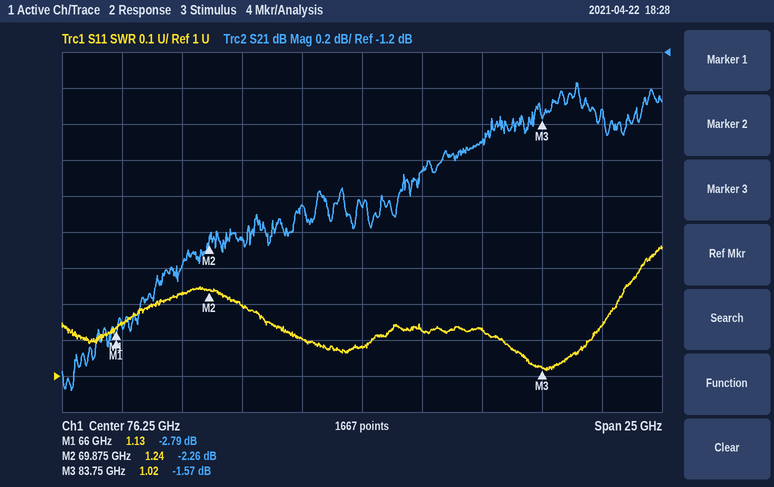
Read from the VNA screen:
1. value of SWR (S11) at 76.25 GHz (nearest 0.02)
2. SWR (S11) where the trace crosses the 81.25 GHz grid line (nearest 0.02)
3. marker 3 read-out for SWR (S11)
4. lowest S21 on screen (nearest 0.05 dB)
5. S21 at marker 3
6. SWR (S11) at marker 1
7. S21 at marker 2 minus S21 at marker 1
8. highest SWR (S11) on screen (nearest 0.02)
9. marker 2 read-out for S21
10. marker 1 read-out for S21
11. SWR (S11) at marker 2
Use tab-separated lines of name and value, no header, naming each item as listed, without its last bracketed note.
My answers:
value of SWR (S11) at 76.25 GHz	1.08
SWR (S11) where the trace crosses the 81.25 GHz grid line	1.14
marker 3 read-out for SWR	1.02
lowest S21 on screen	-3.10 dB
S21 at marker 3	-1.57 dB
SWR (S11) at marker 1	1.13
S21 at marker 2 minus S21 at marker 1	0.53 dB
highest SWR (S11) on screen	1.36
marker 2 read-out for S21	-2.26 dB
marker 1 read-out for S21	-2.79 dB
SWR (S11) at marker 2	1.24
